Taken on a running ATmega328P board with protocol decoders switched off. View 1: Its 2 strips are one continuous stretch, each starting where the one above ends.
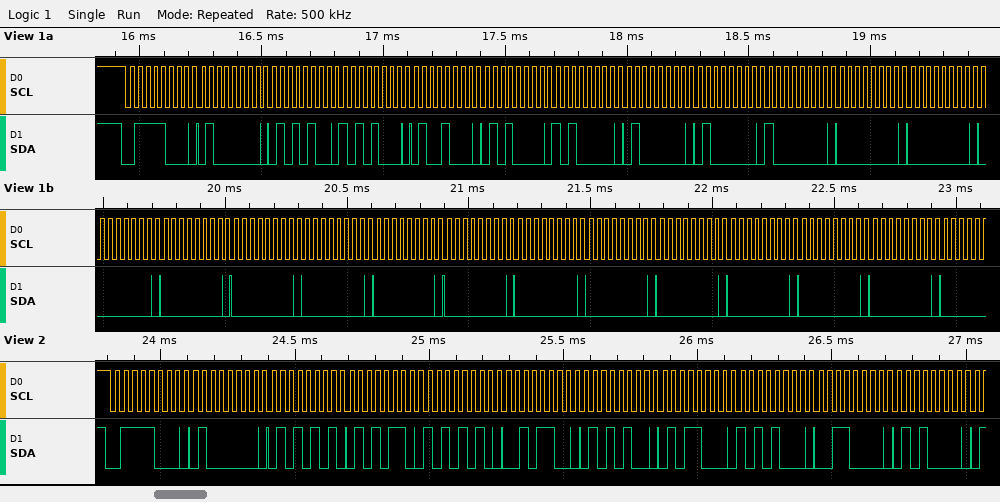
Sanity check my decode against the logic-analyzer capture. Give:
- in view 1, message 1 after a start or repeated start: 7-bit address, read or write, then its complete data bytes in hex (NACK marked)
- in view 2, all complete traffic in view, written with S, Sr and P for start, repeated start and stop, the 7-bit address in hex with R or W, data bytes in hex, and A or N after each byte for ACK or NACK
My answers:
0x3C write: 40 54 A8 48 50 A0 40 40 80 00 00 00 00 00 00 00 00 00 00 00 00 00 00
S 3CW A 40 A 55 A 56 A AA A 2C A 54 A 58 A A8 A 30 A 50 A
